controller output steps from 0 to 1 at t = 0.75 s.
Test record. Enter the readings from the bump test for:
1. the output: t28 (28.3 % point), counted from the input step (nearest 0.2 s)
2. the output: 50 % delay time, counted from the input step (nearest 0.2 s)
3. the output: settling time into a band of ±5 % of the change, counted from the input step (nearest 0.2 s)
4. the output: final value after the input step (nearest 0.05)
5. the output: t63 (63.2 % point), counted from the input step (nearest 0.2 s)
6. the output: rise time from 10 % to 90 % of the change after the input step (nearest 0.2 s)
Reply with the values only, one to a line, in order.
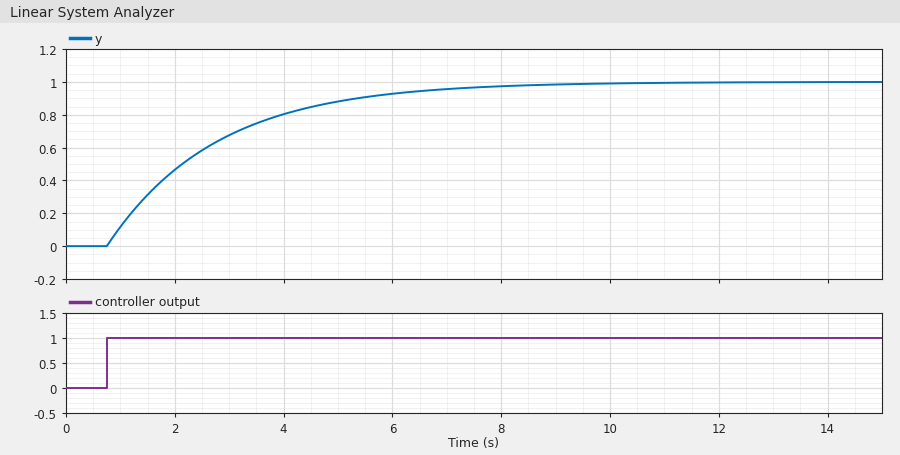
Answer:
0.6 s
1.4 s
6.0 s
1.00
2.0 s
4.4 s
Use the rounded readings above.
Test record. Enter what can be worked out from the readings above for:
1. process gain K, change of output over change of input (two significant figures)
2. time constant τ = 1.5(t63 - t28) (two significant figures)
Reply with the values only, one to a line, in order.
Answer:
1.0
2.1 s
